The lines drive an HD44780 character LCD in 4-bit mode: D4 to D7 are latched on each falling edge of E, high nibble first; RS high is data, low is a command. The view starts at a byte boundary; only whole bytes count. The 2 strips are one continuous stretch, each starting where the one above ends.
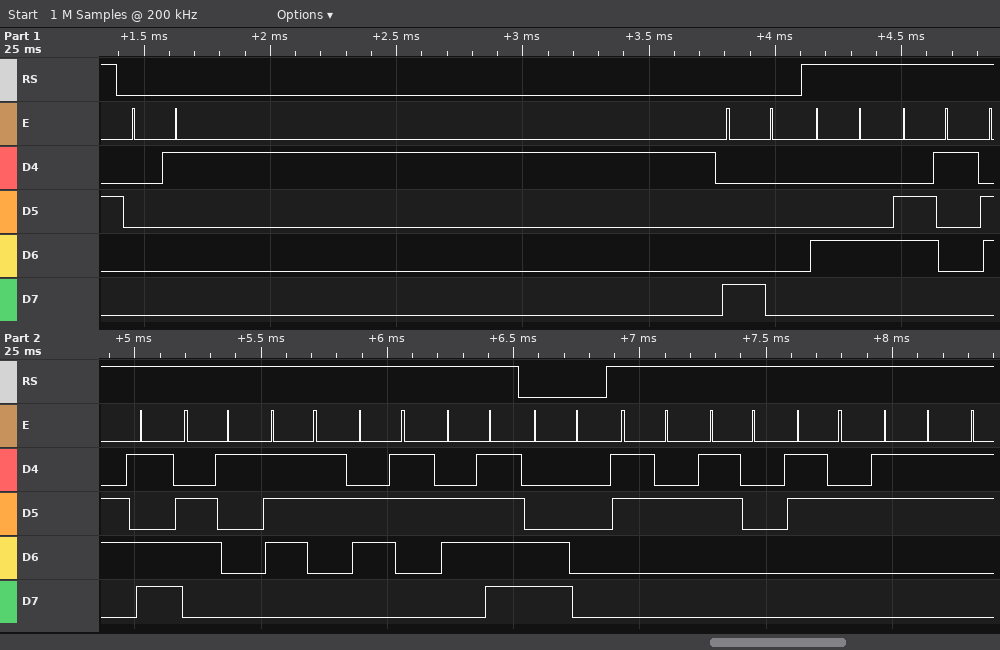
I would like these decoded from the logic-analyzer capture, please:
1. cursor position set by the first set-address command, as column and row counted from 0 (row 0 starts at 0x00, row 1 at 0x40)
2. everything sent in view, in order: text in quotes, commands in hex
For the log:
column 0, row 0
0x01 0x80 "Damasco" 0xC0 "2023"
